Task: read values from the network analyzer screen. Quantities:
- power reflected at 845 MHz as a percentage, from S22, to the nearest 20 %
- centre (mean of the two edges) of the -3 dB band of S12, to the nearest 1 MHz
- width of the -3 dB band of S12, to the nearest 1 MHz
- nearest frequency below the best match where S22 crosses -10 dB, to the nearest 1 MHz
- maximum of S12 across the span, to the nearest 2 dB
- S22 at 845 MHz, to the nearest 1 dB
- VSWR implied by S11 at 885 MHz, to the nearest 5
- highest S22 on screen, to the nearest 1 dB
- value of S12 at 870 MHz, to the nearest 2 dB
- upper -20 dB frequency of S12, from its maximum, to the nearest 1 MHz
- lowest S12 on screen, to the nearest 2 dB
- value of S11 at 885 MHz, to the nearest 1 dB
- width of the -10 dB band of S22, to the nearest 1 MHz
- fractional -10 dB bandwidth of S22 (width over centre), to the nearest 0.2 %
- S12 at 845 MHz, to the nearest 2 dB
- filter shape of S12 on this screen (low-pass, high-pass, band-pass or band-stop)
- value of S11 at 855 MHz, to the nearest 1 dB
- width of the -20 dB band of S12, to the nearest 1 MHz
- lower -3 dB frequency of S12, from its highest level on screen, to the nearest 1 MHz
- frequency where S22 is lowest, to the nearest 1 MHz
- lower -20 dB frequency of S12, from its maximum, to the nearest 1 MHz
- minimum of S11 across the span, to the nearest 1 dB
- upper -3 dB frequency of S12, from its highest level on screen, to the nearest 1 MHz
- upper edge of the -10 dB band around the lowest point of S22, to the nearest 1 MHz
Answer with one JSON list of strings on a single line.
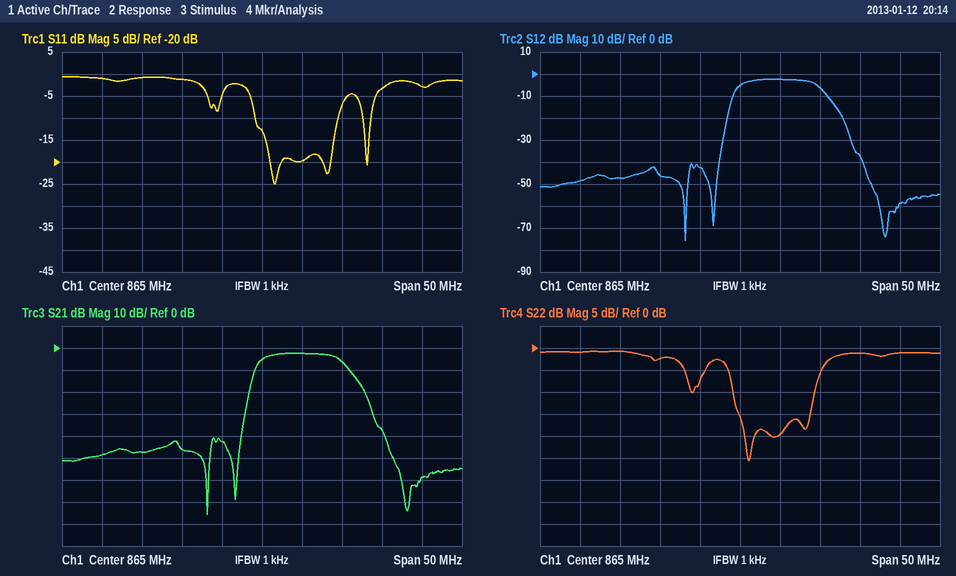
["80 %", "870 MHz", "10 MHz", "864 MHz", "-2 dB", "-1 dB", "5", "-1 dB", "-2 dB", "878 MHz", "-76 dB", "-3 dB", "10 MHz", "1.2 %", "-48 dB", "band-pass", "-1 dB", "15 MHz", "865 MHz", "866 MHz", "863 MHz", "-25 dB", "875 MHz", "874 MHz"]
